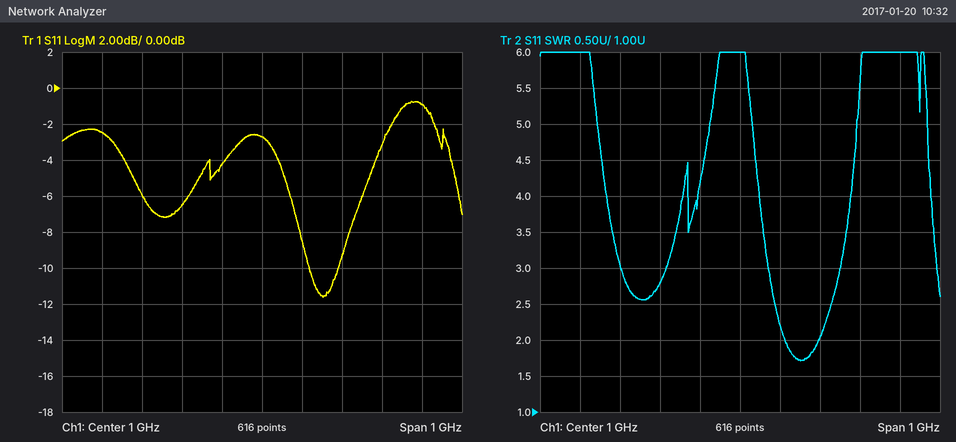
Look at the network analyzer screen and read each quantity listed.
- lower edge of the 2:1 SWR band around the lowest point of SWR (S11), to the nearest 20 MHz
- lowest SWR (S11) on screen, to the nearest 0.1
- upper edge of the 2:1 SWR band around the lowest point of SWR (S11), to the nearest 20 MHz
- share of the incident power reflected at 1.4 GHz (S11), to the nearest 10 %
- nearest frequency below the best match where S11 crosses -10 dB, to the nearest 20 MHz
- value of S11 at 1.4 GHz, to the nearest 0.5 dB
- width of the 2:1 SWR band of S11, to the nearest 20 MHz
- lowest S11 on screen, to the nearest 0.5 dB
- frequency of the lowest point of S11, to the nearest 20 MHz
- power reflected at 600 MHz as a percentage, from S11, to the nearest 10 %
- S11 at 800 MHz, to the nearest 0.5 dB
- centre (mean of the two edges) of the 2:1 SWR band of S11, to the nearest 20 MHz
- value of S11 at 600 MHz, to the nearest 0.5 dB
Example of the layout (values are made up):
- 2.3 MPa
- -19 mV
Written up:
- 1.12 GHz
- 1.7
- 1.20 GHz
- 80 %
- 1.12 GHz
- -1.0 dB
- 80 MHz
- -11.5 dB
- 1.16 GHz
- 60 %
- -6.5 dB
- 1.16 GHz
- -2.5 dB
